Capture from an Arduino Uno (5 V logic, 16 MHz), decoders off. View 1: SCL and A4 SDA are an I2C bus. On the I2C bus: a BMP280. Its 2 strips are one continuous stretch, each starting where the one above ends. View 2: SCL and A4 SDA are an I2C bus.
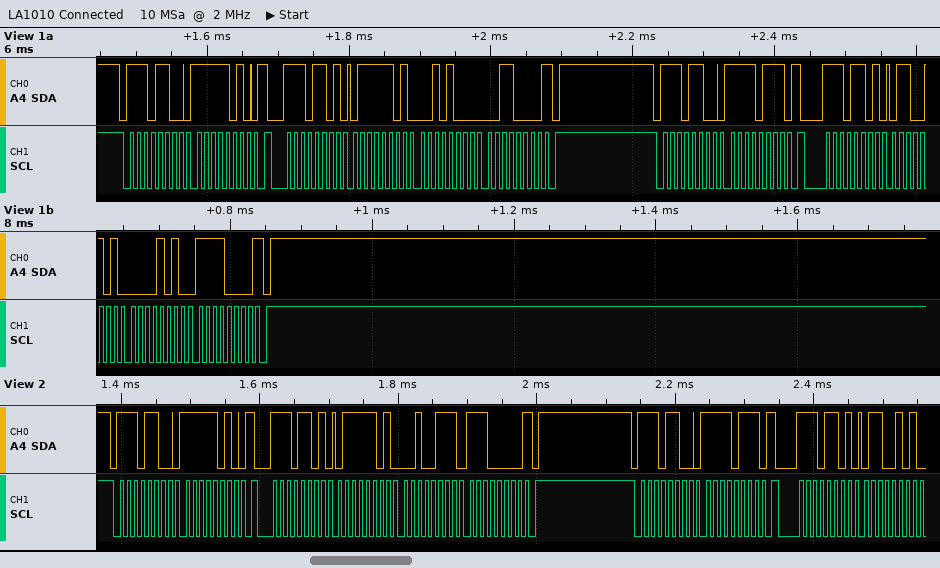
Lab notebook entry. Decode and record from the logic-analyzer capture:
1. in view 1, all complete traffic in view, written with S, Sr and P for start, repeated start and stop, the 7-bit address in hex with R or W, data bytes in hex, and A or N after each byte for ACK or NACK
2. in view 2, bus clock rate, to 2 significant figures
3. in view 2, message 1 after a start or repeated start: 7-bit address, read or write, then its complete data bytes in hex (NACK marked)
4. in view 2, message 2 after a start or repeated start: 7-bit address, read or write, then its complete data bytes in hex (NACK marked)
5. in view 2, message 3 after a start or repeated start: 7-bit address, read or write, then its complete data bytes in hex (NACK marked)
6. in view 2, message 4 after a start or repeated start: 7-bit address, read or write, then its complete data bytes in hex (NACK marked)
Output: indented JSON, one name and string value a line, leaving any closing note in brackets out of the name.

{
  "in view 1, all complete traffic in view, written with S, Sr and P for start, repeated start and stop, the 7-bit address in hex with R or W, data bytes in hex, and A or N after each byte for ACK or NACK": "S 76W A FA A Sr 76R A 7D A 28 A 30 N P S 76W A F7 A Sr 76R A 65 A 0A A F0 N P",
  "in view 2, bus clock rate, to 2 significant figures": "100 kHz",
  "in view 2, message 1 after a start or repeated start: 7-bit address, read or write, then its complete data bytes in hex": "0x76 write: FA",
  "in view 2, message 2 after a start or repeated start: 7-bit address, read or write, then its complete data bytes in hex": "0x76 read: 7D 27 E0 NACK",
  "in view 2, message 3 after a start or repeated start: 7-bit address, read or write, then its complete data bytes in hex": "0x76 write: F7",
  "in view 2, message 4 after a start or repeated start: 7-bit address, read or write, then its complete data bytes in hex": "0x76 read: 65"
}
